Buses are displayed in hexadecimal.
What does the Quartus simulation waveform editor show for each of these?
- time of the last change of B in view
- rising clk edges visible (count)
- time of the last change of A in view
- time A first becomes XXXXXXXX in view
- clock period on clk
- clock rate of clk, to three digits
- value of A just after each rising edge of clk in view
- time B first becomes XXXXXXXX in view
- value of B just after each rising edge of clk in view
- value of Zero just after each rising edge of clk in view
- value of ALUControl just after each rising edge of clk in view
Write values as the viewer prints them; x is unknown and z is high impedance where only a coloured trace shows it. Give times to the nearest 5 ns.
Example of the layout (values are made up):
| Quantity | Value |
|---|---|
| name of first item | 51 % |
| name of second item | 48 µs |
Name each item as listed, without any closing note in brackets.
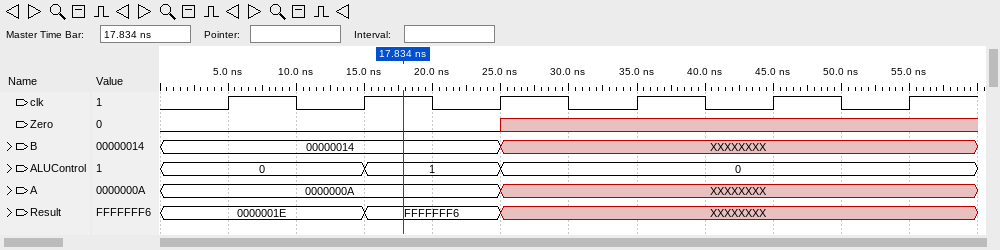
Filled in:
| Quantity | Value |
|---|---|
| time of the last change of B in view | 25 ns |
| rising clk edges visible | 6 |
| time of the last change of A in view | 25 ns |
| time A first becomes XXXXXXXX in view | 25 ns |
| clock period on clk | 10 ns |
| clock rate of clk, to three digits | 100 MHz |
| value of A just after each rising edge of clk in view | 0000000A, 0000000A, XXXXXXXX, XXXXXXXX, XXXXXXXX, XXXXXXXX |
| time B first becomes XXXXXXXX in view | 25 ns |
| value of B just after each rising edge of clk in view | 00000014, 00000014, XXXXXXXX, XXXXXXXX, XXXXXXXX, XXXXXXXX |
| value of Zero just after each rising edge of clk in view | 0 0 x x x x |
| value of ALUControl just after each rising edge of clk in view | 0, 1, 0, 0, 0, 0 |
